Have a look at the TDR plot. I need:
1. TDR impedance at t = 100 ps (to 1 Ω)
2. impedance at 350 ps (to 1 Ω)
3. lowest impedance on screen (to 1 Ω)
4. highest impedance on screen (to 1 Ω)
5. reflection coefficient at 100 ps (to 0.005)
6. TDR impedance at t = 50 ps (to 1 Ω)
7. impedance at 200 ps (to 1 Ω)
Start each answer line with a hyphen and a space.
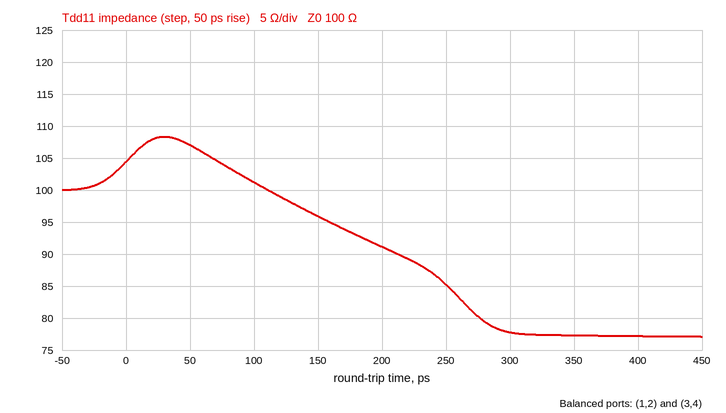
- 101 Ω
- 77 Ω
- 77 Ω
- 108 Ω
- +0.005
- 107 Ω
- 91 Ω
